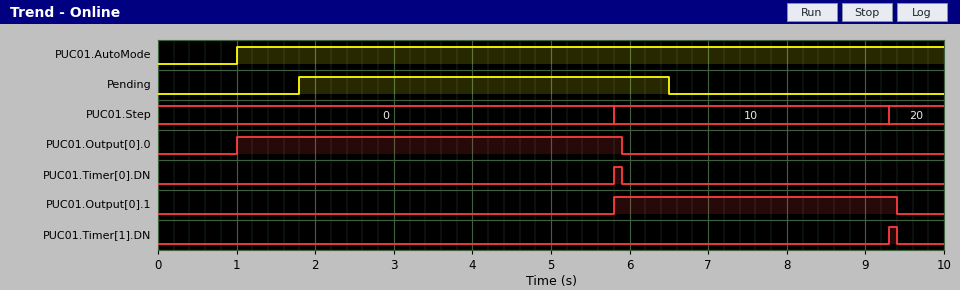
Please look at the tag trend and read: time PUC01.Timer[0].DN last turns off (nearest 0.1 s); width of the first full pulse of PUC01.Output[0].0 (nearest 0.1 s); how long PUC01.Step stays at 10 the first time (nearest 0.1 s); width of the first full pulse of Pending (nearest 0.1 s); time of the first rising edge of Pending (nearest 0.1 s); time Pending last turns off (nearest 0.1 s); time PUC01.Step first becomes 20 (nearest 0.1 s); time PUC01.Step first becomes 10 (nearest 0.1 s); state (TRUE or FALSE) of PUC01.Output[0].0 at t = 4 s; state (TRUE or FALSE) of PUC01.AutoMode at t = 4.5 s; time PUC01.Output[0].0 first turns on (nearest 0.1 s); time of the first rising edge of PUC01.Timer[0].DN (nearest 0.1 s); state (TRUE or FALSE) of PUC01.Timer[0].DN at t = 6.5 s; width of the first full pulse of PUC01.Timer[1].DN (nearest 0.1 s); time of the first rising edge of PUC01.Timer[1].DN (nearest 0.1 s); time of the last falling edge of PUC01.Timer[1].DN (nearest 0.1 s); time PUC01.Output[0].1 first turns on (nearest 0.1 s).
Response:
5.9 s
4.9 s
3.5 s
4.7 s
1.8 s
6.5 s
9.3 s
5.8 s
TRUE
TRUE
1.0 s
5.8 s
FALSE
0.1 s
9.3 s
9.4 s
5.8 s
